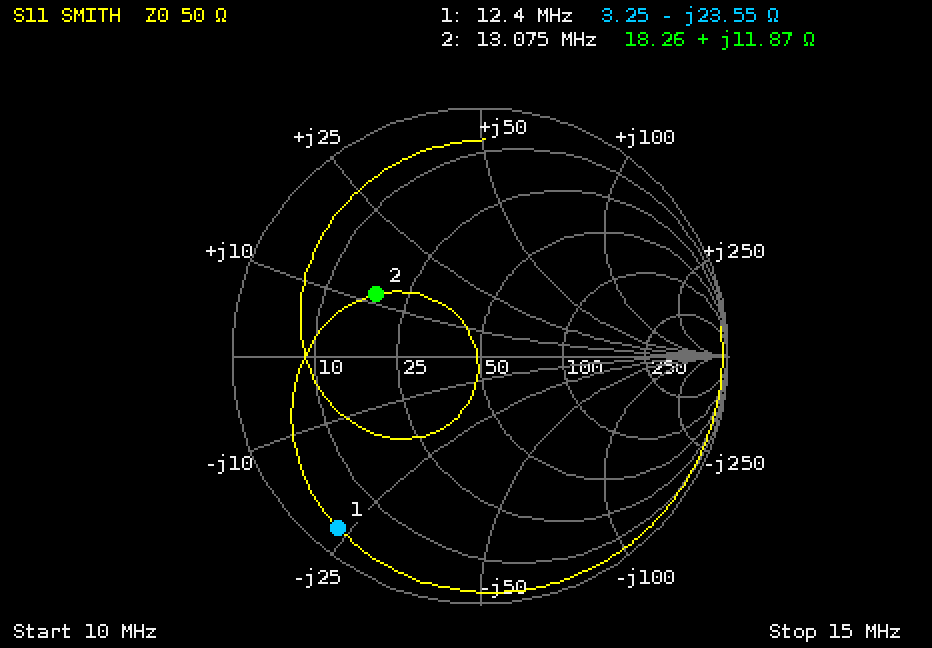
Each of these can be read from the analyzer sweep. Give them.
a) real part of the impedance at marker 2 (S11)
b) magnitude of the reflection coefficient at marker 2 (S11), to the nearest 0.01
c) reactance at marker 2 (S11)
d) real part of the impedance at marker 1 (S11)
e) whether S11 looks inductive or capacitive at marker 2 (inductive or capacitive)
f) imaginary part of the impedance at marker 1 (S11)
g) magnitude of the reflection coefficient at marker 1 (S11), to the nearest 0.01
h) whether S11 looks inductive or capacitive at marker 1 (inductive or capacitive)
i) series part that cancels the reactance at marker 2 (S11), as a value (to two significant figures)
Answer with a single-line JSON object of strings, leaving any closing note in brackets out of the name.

{"real part of the impedance at marker 2": "18.26 Ω", "magnitude of the reflection coefficient at marker 2 (S11), to the nearest 0.01": "0.49", "reactance at marker 2": "+11.87 Ω", "real part of the impedance at marker 1": "3.25 Ω", "whether S11 looks inductive or capacitive at marker 2": "inductive", "imaginary part of the impedance at marker 1": "-23.55 Ω", "magnitude of the reflection coefficient at marker 1 (S11), to the nearest 0.01": "0.90", "whether S11 looks inductive or capacitive at marker 1": "capacitive", "series part that cancels the reactance at marker 2 (S11), as a value": "1.0 nF"}
